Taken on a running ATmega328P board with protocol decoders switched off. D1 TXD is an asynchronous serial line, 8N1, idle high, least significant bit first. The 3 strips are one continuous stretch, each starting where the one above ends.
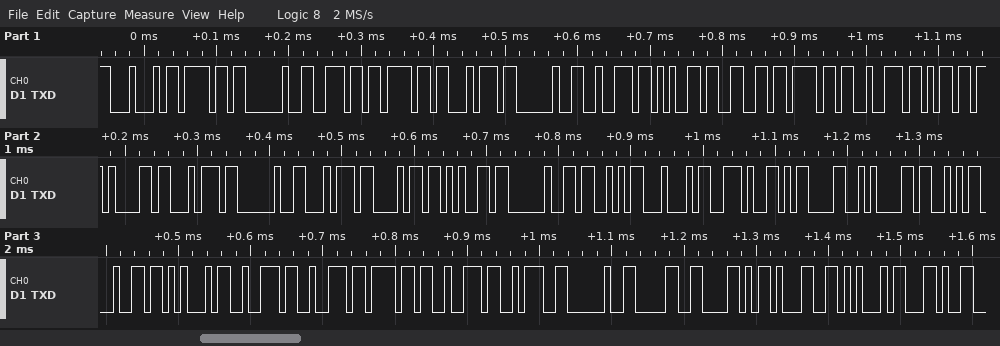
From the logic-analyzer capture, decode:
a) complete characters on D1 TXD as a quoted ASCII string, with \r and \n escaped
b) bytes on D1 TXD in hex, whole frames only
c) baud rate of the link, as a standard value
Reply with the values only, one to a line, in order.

"Do not reformat the SD.\r\nSdError: 0X1E,"
0x44 0x6F 0x20 0x6E 0x6F 0x74 0x20 0x72 0x65 0x66 0x6F 0x72 0x6D 0x61 0x74 0x20 0x74 0x68 0x65 0x20 0x53 0x44 0x2E 0x0D 0x0A 0x53 0x64 0x45 0x72 0x72 0x6F 0x72 0x3A 0x20 0x30 0x58 0x31 0x45 0x2C
115200 baud
